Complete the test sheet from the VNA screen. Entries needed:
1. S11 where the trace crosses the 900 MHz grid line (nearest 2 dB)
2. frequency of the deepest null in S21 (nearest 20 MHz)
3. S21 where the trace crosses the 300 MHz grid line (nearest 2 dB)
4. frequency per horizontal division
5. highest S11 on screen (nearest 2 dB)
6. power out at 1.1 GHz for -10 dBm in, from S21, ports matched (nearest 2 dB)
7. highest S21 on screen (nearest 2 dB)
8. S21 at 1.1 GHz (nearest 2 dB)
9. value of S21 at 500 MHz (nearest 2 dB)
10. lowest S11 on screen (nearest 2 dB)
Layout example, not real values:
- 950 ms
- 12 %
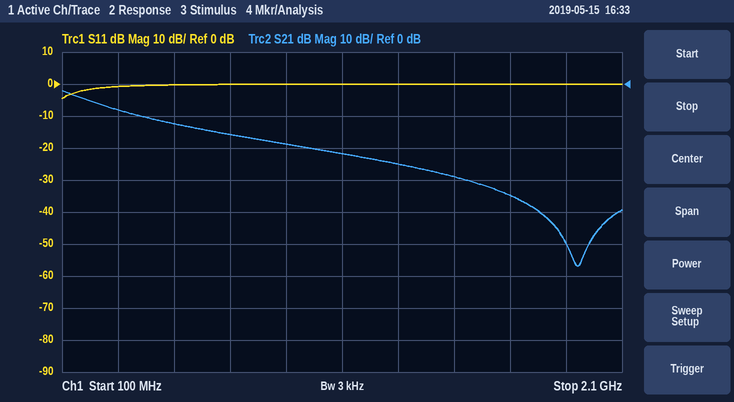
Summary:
- 0 dB
- 1.94 GHz
- -8 dB
- 200 MHz
- 0 dB
- -32 dBm
- -2 dB
- -22 dB
- -12 dB
- -4 dB
